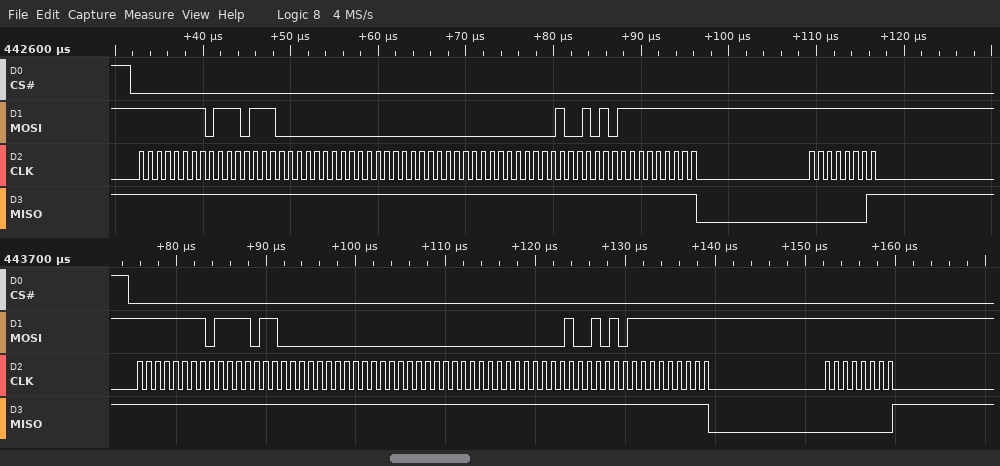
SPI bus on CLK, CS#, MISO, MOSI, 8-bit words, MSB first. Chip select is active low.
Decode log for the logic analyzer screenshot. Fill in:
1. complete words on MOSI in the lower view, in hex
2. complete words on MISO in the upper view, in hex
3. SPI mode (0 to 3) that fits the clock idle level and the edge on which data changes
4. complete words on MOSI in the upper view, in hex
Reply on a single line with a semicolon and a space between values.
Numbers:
FF, 7B, 00, 00, 00, 00, 95, FF, FF; FF, FF, FF, FF, FF, FF, FF, FF, 01; 0; FF, 77, 00, 00, 00, 00, 95, FF, FF
